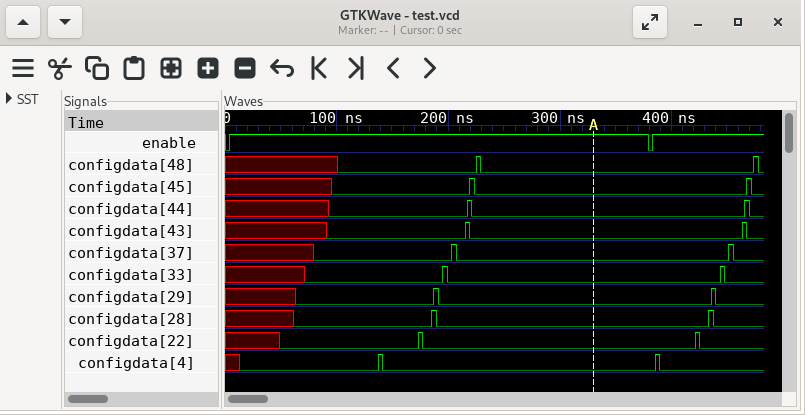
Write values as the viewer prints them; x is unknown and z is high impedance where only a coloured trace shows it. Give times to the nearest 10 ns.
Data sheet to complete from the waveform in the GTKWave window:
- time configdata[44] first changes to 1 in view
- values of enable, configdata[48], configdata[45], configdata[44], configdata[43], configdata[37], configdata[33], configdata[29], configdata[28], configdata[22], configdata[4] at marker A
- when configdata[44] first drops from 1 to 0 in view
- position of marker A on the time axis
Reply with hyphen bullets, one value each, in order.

- 220 ns
- enable=1, configdata[48]=0, configdata[45]=0, configdata[44]=0, configdata[43]=0, configdata[37]=0, configdata[33]=0, configdata[29]=0, configdata[28]=0, configdata[22]=0, configdata[4]=0
- 220 ns
- 330 ns
